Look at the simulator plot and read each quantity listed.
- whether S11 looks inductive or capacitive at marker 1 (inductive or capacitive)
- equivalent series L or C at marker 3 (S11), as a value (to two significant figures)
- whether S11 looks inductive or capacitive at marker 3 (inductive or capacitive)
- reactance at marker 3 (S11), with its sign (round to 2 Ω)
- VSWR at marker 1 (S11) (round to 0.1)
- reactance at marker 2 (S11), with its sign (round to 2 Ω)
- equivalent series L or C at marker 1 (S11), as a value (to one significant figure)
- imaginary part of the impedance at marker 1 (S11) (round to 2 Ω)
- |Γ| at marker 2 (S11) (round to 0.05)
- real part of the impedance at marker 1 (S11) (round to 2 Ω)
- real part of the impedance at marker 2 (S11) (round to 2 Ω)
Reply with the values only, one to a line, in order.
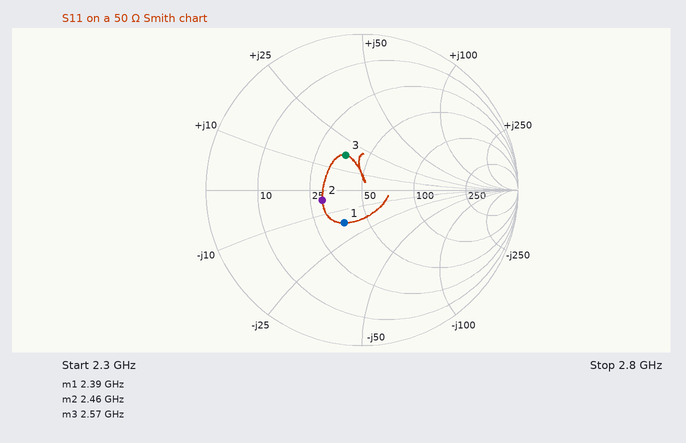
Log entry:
capacitive
1.1 nH
inductive
+18 Ω
1.6
-4 Ω
4 pF
-16 Ω
0.25
36 Ω
30 Ω
